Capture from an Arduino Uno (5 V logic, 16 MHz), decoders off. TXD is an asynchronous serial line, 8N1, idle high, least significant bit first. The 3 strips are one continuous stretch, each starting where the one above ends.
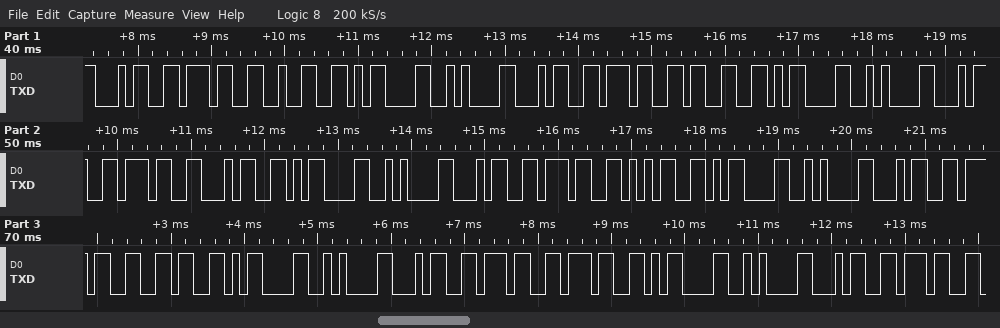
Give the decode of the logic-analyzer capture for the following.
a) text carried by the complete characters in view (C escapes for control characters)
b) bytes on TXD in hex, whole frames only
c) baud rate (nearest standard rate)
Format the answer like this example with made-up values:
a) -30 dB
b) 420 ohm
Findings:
a) "472\r\n473\r\n474\r\n475\r\n476\r\n477\r\n47"
b) 34 37 32 0D 0A 34 37 33 0D 0A 34 37 34 0D 0A 34 37 35 0D 0A 34 37 36 0D 0A 34 37 37 0D 0A 34 37
c) 9600 baud
